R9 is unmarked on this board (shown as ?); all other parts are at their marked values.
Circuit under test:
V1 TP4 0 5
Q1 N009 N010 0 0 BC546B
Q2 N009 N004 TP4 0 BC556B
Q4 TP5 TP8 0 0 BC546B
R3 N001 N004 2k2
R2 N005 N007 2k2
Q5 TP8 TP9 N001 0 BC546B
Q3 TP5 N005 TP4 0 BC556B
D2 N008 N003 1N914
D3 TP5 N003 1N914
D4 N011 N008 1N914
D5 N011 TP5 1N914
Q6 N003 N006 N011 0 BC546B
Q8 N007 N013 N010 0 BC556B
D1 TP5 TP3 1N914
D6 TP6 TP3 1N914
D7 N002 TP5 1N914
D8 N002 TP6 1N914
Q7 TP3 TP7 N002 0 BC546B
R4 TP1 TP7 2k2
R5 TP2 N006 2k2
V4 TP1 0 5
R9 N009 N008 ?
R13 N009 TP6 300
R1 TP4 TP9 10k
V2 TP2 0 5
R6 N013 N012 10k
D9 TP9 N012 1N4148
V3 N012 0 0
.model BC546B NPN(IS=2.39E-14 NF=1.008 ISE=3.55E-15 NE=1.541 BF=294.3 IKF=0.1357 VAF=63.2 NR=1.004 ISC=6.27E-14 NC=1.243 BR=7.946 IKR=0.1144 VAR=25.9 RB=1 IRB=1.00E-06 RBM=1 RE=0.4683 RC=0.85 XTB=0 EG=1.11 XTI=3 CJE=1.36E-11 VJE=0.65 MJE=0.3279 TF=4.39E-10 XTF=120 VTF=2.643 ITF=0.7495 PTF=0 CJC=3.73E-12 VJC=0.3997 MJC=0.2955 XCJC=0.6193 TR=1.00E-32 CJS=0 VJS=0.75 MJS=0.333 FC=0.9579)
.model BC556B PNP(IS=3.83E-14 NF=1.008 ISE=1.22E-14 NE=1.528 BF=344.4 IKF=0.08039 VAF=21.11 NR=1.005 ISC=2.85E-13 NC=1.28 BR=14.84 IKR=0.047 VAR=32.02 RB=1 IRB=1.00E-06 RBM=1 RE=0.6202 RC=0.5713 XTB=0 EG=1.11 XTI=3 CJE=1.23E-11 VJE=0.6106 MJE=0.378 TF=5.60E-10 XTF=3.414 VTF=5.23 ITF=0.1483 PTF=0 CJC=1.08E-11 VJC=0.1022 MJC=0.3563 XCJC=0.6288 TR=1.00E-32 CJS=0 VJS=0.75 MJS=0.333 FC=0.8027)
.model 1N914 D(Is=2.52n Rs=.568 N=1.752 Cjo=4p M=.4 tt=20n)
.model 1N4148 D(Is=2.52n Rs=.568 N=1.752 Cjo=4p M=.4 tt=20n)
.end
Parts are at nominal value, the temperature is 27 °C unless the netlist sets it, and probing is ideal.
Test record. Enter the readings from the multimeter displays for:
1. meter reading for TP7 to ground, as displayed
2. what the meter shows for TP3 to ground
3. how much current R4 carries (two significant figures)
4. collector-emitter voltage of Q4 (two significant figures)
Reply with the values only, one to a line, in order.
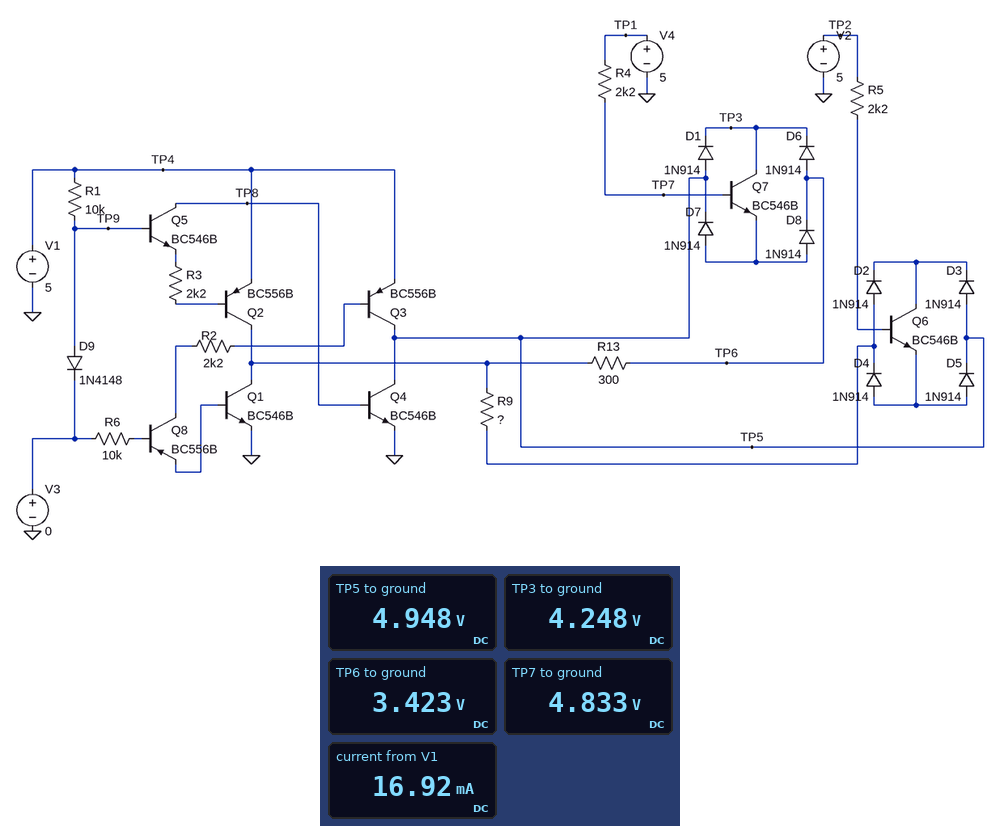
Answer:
4.833 V
4.248 V
76 µA
4.9 V
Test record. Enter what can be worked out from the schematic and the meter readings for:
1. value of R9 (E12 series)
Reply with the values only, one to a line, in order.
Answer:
820 Ω
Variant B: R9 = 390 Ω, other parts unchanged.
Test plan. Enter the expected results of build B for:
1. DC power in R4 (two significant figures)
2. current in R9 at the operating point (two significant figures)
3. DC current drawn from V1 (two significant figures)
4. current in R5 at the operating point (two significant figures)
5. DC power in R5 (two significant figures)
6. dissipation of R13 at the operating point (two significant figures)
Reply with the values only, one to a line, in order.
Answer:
14 µW
8.7 mA
21 mA
72 µA
11 µW
37 mW
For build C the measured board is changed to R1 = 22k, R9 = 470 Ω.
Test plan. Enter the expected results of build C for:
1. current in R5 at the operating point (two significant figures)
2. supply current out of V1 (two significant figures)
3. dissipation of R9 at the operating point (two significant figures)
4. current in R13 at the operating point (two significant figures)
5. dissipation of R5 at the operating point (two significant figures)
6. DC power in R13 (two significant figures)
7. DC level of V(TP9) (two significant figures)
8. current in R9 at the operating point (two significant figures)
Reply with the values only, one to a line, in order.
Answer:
66 µA
20 mA
25 mW
11 mA
9.6 µW
37 mW
510 mV
7.3 mA
